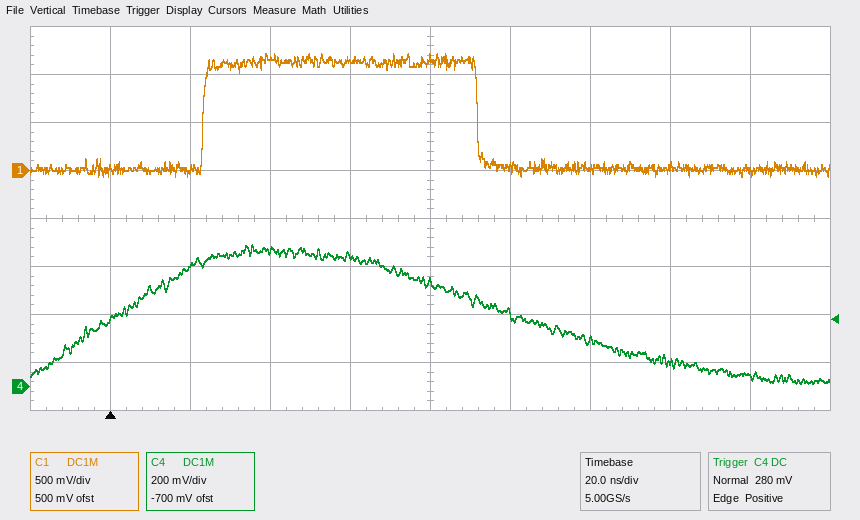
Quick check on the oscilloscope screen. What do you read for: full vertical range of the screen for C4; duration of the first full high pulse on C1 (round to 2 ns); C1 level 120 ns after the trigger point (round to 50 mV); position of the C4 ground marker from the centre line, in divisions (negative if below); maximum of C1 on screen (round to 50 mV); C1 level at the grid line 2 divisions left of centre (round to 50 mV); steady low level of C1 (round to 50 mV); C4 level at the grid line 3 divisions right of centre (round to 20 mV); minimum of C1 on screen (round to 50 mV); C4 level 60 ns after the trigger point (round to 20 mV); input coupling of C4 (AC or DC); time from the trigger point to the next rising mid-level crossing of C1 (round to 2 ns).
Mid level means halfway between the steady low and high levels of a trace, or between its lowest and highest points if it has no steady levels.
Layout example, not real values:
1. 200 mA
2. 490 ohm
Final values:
1. 1.6 V
2. 68 ns
3. 0 mV
4. -3.5 div
5. 1.20 V
6. 1.20 V
7. 0 mV
8. 100 mV
9. -50 mV
10. 540 mV
11. DC
12. 24 ns
